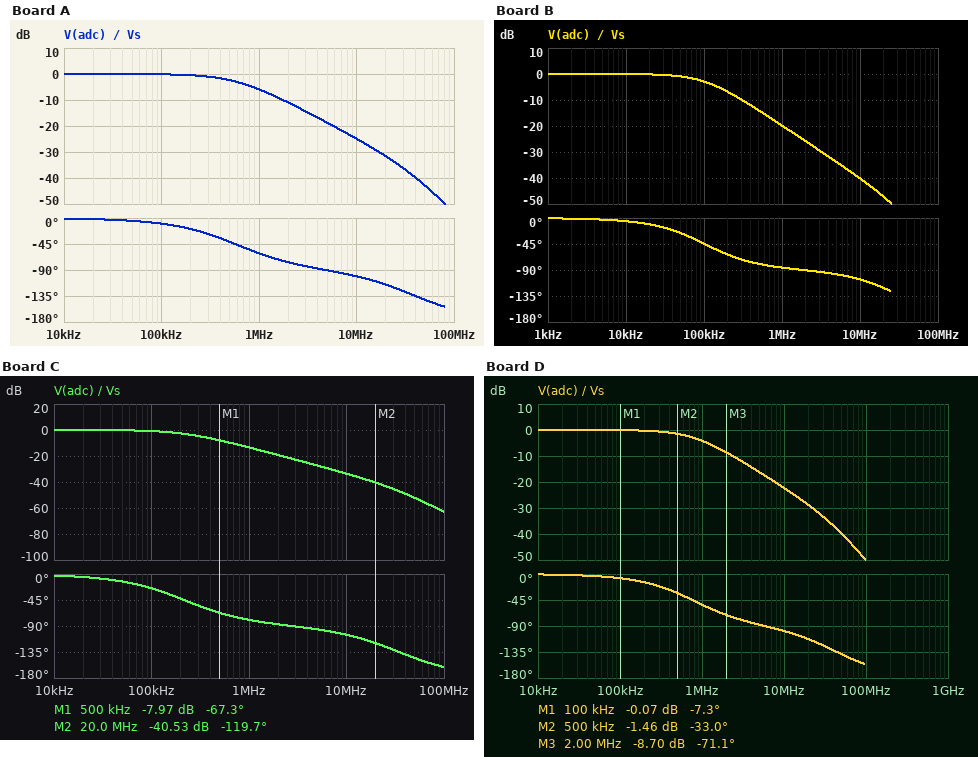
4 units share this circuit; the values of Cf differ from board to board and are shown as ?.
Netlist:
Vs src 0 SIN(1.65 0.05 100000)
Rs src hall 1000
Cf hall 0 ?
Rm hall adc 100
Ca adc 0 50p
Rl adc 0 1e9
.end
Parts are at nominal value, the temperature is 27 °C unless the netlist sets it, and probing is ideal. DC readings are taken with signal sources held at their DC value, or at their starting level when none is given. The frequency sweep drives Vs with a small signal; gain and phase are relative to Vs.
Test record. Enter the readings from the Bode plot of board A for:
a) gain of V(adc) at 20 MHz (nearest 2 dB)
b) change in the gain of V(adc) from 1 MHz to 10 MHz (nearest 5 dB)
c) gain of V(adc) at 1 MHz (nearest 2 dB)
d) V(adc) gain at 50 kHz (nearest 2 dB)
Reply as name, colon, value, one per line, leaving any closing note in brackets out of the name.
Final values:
gain of V(adc) at 20 MHz: -32 dB
change in the gain of V(adc) from 1 MHz to 10 MHz: -20 dB
gain of V(adc) at 1 MHz: -6 dB
V(adc) gain at 50 kHz: 0 dB
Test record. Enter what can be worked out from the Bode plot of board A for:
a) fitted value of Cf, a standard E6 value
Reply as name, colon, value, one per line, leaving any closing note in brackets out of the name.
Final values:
fitted value of Cf, a standard E6 value: 220 pF
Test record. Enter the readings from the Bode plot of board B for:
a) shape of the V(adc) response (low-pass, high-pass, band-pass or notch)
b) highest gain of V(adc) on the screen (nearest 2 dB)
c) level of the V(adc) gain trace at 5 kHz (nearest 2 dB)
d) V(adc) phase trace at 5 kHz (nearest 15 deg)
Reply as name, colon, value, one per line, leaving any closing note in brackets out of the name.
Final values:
shape of the V(adc) response: low-pass
highest gain of V(adc) on the screen: 0 dB
level of the V(adc) gain trace at 5 kHz: 0 dB
V(adc) phase trace at 5 kHz: 0 deg
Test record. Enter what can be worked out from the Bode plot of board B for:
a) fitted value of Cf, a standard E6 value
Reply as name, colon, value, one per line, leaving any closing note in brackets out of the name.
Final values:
fitted value of Cf, a standard E6 value: 1.5 nF
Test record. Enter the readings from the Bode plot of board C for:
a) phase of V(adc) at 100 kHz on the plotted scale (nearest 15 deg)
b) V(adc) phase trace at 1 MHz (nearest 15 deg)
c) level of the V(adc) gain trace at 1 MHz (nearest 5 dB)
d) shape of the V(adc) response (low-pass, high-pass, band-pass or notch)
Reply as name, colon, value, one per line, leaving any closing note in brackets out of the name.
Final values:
phase of V(adc) at 100 kHz on the plotted scale: -30 deg
V(adc) phase trace at 1 MHz: -75 deg
level of the V(adc) gain trace at 1 MHz: -15 dB
shape of the V(adc) response: low-pass
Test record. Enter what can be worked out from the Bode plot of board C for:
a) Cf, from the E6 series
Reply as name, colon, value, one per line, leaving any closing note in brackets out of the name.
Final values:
Cf, from the E6 series: 680 pF
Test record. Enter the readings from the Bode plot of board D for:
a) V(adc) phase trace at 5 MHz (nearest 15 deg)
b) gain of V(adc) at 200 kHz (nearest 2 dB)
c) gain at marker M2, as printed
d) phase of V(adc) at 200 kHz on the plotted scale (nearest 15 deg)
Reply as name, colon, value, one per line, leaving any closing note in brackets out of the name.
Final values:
V(adc) phase trace at 5 MHz: -90 deg
gain of V(adc) at 200 kHz: 0 dB
gain at marker M2, as printed: -1.46 dB
phase of V(adc) at 200 kHz on the plotted scale: -15 deg
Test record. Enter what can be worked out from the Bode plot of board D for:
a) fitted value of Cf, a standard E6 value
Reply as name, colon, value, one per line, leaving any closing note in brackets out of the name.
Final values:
fitted value of Cf, a standard E6 value: 150 pF
